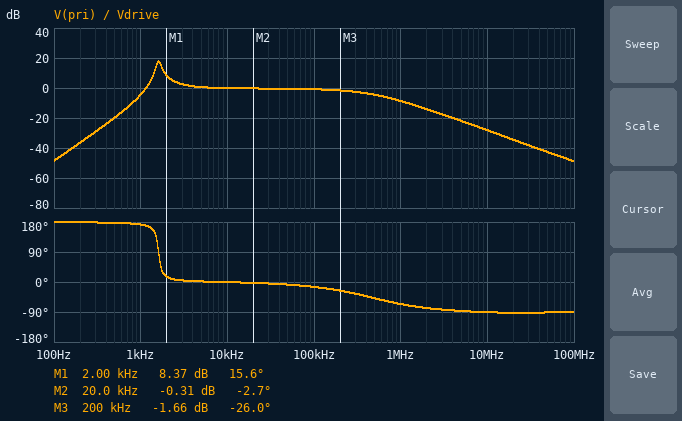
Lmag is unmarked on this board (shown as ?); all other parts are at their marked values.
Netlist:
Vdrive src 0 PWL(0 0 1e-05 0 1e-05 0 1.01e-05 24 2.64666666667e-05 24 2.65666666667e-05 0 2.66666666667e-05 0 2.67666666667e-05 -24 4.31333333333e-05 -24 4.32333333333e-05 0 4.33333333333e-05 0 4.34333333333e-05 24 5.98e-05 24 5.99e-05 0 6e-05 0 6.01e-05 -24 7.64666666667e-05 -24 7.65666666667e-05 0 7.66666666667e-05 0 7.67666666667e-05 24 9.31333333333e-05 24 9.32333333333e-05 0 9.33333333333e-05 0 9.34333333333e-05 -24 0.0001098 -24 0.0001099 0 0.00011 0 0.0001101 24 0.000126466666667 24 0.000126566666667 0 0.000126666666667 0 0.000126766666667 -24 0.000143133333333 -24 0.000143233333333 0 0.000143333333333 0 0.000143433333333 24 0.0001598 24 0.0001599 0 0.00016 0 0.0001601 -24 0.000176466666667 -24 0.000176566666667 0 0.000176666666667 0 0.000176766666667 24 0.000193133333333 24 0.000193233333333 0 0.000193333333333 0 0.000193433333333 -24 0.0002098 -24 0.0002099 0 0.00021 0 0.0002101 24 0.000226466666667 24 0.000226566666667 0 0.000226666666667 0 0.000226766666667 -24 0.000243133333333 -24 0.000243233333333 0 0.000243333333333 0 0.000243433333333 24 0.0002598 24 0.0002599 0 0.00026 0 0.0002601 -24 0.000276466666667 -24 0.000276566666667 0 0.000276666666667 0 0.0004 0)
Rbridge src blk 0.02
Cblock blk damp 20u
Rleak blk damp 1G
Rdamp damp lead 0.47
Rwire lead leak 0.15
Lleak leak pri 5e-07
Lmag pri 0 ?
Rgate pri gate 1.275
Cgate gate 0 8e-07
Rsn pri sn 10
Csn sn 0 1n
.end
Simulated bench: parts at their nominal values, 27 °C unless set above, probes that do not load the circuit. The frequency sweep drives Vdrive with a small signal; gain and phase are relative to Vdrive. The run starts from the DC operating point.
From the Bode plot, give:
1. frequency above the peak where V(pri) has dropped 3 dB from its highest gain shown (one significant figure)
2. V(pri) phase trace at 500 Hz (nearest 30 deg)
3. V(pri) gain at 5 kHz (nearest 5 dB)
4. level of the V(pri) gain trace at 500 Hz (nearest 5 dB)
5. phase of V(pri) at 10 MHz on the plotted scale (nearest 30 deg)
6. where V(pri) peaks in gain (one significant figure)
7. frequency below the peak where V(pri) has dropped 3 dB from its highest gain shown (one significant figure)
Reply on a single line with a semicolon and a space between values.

2 kHz; 180 deg; 0 dB; -20 dB; -90 deg; 2 kHz; 2 kHz
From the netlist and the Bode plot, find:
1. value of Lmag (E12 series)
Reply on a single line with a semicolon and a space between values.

470 µH
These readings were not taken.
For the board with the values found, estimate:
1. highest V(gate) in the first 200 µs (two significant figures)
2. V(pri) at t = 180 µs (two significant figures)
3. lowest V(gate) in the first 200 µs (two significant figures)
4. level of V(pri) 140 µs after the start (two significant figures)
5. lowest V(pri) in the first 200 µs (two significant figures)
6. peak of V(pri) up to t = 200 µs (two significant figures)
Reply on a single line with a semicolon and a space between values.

23 V; 21 V; -25 V; -25 V; -25 V; 23 V
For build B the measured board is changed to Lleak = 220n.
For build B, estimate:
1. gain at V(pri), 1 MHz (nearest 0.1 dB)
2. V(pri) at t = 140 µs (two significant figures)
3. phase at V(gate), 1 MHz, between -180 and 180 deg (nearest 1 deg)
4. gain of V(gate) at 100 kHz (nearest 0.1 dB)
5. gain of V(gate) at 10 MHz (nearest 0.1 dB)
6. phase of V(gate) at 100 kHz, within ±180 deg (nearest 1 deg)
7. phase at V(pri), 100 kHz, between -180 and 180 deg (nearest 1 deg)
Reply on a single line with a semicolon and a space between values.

-4.8 dB; -25 V; -122 deg; -2.7 dB; -57.2 dB; -45 deg; -12 deg
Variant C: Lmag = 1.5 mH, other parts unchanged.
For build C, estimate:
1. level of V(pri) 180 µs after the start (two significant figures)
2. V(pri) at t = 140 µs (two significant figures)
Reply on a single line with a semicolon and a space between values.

22 V; -24 V
